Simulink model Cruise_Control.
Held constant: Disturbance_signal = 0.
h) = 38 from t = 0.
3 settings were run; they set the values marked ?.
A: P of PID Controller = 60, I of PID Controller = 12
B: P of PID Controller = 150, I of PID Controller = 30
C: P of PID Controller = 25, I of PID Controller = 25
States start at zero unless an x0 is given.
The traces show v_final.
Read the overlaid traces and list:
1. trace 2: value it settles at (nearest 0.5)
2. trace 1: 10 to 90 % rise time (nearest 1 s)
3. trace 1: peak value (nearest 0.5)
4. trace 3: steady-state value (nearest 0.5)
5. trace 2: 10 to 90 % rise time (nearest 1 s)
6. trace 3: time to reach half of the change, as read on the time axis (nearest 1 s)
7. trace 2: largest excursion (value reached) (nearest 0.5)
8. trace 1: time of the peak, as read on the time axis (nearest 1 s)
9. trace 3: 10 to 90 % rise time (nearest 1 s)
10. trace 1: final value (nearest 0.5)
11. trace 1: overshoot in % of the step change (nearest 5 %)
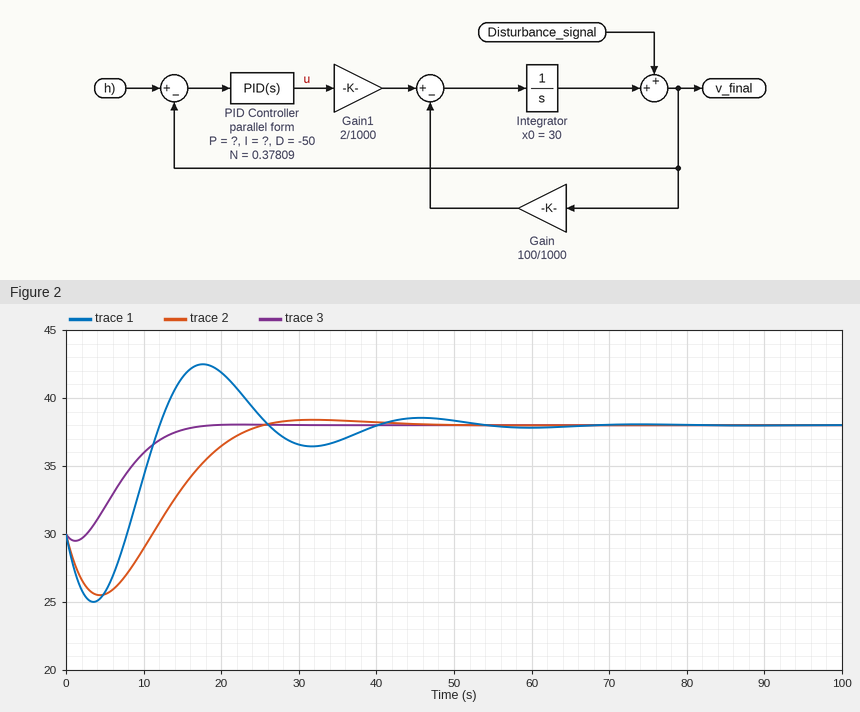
38.0
3 s
42.5
38.0
10 s
7 s
38.5
18 s
9 s
38.0
55 %
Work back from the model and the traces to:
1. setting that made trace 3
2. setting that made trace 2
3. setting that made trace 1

B
A
C
